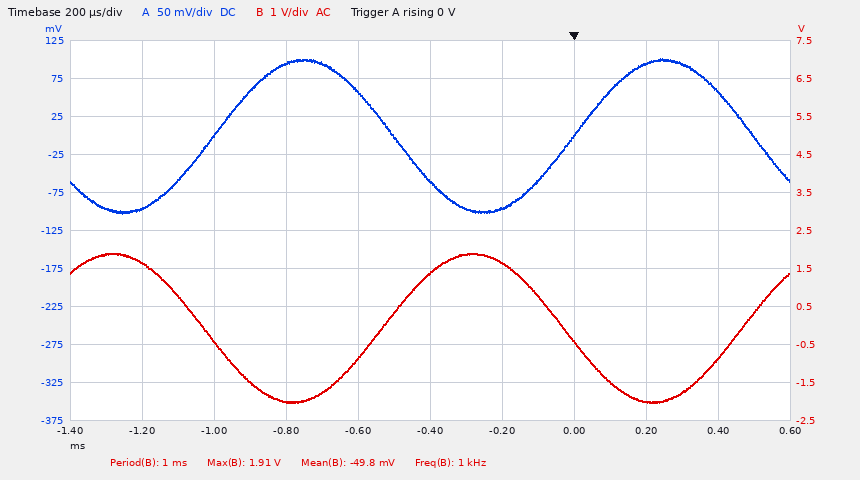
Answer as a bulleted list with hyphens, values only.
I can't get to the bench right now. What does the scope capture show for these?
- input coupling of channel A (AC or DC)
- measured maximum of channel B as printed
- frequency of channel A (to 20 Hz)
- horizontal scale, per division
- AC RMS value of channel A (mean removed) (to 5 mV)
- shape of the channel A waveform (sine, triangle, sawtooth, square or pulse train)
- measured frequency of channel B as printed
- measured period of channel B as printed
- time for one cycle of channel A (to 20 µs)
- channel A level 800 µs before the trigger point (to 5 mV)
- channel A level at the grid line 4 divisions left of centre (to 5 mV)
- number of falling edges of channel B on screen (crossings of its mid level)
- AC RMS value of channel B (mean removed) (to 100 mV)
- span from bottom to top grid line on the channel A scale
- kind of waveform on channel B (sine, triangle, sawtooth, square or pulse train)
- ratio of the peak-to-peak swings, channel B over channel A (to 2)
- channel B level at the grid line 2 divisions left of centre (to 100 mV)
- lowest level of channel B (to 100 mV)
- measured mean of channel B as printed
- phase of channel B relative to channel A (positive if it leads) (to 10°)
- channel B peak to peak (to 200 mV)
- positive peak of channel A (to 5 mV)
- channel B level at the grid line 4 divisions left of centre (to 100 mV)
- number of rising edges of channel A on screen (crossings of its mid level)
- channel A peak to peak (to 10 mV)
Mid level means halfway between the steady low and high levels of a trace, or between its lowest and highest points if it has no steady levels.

- DC
- 1.91 V
- 1.00 kHz
- 200 µs
- 70 mV
- sine
- 1 kHz
- 1 ms
- 1.00 ms
- 95 mV
- -95 mV
- 2
- 1.4 V
- 500 mV
- sine
- 20
- -2.0 V
- -2.0 V
- -49.8 mV
- -170°
- 4.0 V
- 100 mV
- 1.7 V
- 2
- 200 mV
